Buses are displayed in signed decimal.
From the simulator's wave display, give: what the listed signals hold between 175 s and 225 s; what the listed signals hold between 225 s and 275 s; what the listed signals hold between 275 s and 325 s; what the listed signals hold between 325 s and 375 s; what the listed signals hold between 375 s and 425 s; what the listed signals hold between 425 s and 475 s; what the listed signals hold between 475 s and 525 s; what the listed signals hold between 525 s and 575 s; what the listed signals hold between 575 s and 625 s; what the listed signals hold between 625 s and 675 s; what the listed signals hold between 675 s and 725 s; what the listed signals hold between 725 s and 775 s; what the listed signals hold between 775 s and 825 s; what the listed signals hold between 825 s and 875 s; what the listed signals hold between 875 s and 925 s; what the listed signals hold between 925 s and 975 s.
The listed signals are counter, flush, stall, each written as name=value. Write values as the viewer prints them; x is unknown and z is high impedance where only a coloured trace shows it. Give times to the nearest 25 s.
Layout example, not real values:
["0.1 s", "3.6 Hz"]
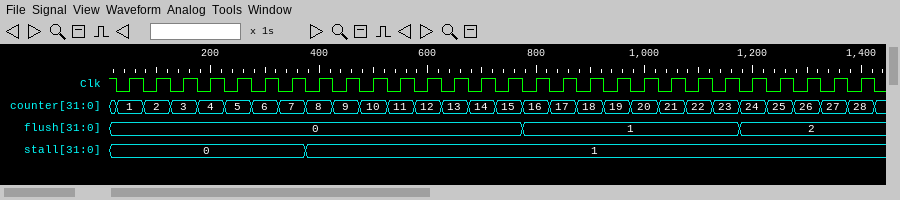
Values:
["counter=4, flush=0, stall=0", "counter=5, flush=0, stall=0", "counter=6, flush=0, stall=0", "counter=7, flush=0, stall=0", "counter=8, flush=0, stall=1", "counter=9, flush=0, stall=1", "counter=10, flush=0, stall=1", "counter=11, flush=0, stall=1", "counter=12, flush=0, stall=1", "counter=13, flush=0, stall=1", "counter=14, flush=0, stall=1", "counter=15, flush=0, stall=1", "counter=16, flush=1, stall=1", "counter=17, flush=1, stall=1", "counter=18, flush=1, stall=1", "counter=19, flush=1, stall=1"]
